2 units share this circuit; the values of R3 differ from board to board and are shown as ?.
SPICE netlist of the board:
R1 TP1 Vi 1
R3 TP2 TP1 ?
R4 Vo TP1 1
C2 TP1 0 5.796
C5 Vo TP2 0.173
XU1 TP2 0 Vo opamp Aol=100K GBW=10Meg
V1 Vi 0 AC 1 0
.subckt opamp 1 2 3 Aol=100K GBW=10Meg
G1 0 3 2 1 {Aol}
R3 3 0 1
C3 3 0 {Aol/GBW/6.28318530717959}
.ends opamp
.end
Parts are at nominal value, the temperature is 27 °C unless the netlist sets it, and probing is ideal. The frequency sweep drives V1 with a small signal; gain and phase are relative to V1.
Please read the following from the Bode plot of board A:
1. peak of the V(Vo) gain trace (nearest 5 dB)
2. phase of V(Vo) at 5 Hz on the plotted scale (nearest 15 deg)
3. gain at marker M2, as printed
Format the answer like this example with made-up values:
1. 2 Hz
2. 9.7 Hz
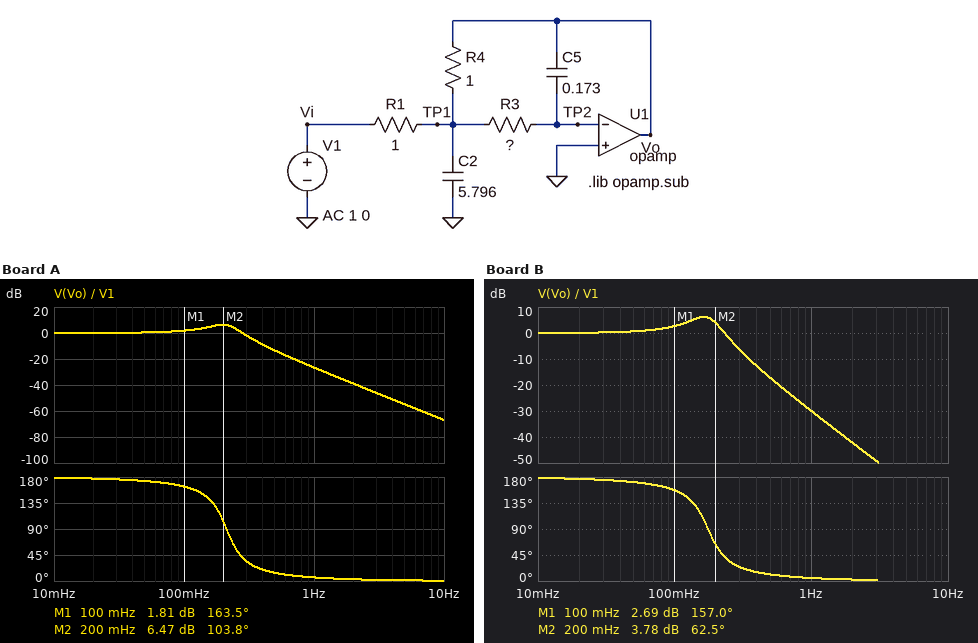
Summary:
1. 5 dB
2. 0 deg
3. 6.47 dB
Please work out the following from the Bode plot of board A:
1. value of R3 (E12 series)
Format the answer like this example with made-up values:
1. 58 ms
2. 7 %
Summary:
1. 0.56 Ω
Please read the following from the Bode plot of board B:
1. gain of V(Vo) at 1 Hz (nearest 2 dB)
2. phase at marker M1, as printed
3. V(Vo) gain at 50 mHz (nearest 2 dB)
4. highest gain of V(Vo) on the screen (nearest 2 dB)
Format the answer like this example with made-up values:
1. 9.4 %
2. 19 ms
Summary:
1. -30 dB
2. 157.0 deg
3. 0 dB
4. 6 dB
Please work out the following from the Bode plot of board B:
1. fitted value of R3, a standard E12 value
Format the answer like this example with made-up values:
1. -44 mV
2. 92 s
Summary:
1. 0.82 Ω
